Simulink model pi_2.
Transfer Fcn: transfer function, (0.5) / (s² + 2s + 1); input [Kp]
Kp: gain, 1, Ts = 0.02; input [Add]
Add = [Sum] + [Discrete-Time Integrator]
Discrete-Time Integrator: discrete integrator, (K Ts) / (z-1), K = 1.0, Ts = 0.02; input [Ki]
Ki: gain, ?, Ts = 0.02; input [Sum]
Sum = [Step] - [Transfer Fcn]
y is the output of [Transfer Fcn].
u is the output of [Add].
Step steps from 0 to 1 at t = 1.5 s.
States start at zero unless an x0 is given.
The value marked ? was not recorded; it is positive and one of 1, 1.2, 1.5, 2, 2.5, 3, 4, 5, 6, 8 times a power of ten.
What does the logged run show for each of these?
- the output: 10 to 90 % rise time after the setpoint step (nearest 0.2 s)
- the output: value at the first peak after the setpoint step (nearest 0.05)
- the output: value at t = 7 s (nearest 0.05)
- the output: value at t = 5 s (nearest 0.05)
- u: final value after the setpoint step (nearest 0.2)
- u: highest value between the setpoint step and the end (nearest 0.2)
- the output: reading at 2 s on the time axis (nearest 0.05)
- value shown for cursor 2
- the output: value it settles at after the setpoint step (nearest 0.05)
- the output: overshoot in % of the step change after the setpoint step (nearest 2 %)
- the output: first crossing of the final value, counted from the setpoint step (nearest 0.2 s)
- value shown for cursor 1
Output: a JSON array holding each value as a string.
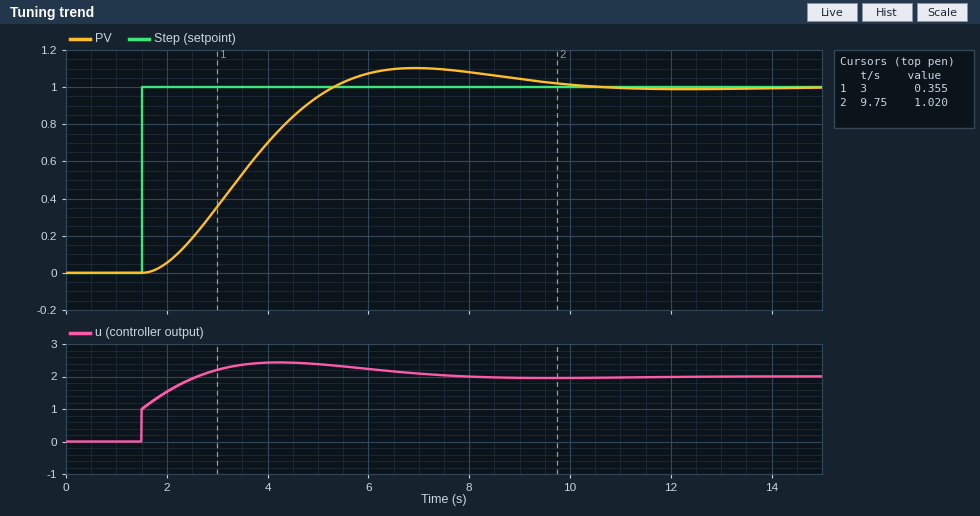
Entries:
["2.6 s", "1.10", "1.10", "0.95", "2.0", "2.4", "0.05", "1.020", "1.00", "10 %", "3.8 s", "0.355"]
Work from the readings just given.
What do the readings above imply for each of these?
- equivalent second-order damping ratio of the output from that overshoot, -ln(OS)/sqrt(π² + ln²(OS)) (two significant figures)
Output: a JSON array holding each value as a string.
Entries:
["0.59"]
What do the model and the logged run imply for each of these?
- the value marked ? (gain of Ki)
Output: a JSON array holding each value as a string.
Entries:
["1.2"]
